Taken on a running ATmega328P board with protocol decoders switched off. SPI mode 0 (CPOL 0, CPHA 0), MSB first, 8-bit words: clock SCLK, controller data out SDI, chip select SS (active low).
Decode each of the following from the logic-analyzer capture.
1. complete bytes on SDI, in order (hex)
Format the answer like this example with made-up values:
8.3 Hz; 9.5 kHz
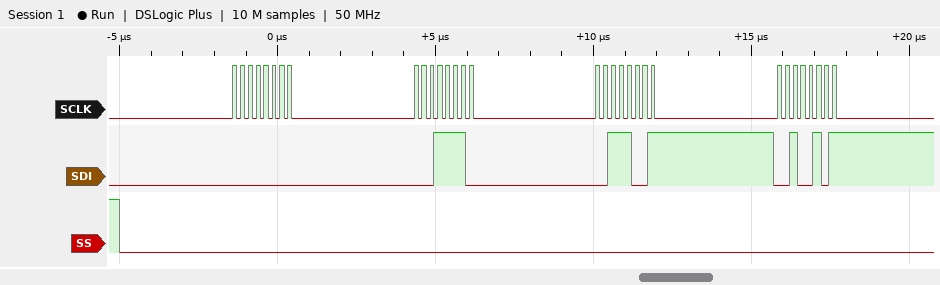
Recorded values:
00 1E 39 25
